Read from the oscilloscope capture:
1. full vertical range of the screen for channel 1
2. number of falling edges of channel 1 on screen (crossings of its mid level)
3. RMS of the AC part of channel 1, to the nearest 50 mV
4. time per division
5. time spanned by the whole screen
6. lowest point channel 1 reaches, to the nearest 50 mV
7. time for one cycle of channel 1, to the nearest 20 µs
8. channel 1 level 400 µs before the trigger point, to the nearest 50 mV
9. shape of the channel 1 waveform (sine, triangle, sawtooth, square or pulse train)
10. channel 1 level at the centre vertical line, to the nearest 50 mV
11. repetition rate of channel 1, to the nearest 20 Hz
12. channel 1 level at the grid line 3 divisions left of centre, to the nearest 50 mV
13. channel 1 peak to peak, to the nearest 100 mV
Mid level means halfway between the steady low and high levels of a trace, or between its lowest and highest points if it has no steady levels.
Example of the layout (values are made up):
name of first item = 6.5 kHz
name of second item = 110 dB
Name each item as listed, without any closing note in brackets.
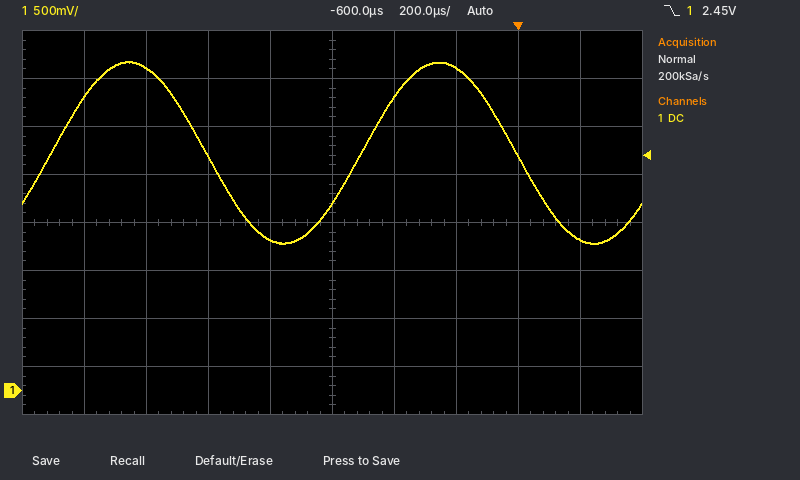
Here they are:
full vertical range of the screen for channel 1 = 4 V
number of falling edges of channel 1 on screen = 2
RMS of the AC part of channel 1, to the nearest 50 mV = 650 mV
time per division = 200 µs
time spanned by the whole screen = 2 ms
lowest point channel 1 reaches, to the nearest 50 mV = 1.55 V
time for one cycle of channel 1, to the nearest 20 µs = 1.00 ms
channel 1 level 400 µs before the trigger point, to the nearest 50 mV = 3.05 V
shape of the channel 1 waveform = sine
channel 1 level at the centre vertical line, to the nearest 50 mV = 1.95 V
repetition rate of channel 1, to the nearest 20 Hz = 1.00 kHz
channel 1 level at the grid line 3 divisions left of centre, to the nearest 50 mV = 3.35 V
channel 1 peak to peak, to the nearest 100 mV = 1.90 V
